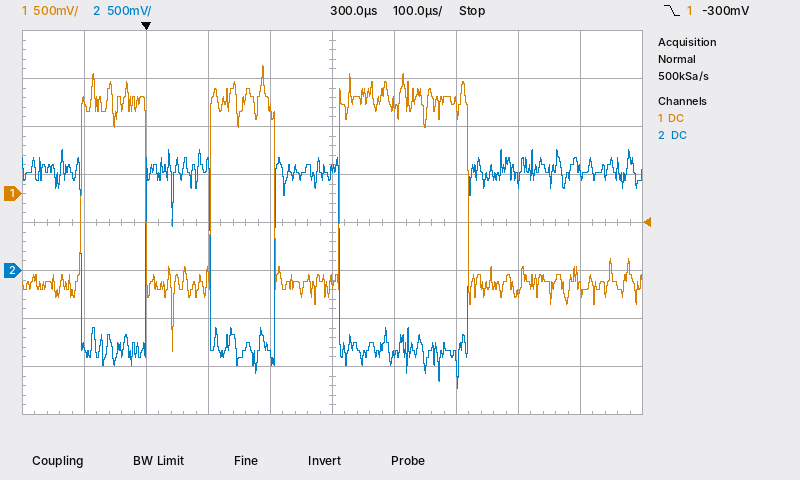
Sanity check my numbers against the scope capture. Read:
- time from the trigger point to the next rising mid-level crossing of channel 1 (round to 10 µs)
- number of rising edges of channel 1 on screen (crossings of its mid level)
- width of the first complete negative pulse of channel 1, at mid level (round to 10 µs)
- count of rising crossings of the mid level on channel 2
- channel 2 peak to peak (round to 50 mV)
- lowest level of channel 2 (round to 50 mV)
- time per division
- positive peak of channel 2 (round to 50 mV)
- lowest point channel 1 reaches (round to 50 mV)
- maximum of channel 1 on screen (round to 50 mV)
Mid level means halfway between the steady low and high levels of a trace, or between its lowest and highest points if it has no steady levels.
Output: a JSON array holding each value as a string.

["100 µs", "3", "100 µs", "3", "2.50 V", "-1.25 V", "100 µs", "1.25 V", "-1.65 V", "1.35 V"]
